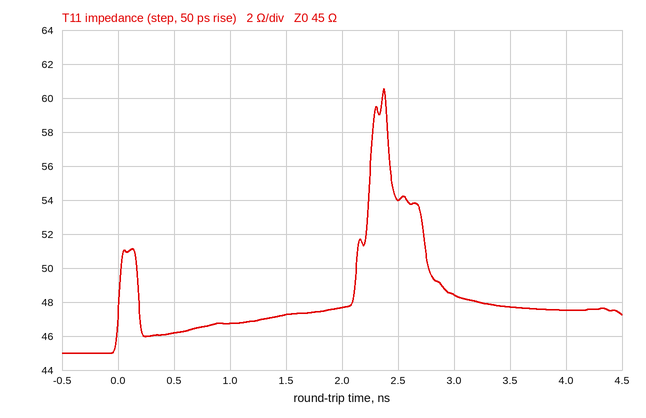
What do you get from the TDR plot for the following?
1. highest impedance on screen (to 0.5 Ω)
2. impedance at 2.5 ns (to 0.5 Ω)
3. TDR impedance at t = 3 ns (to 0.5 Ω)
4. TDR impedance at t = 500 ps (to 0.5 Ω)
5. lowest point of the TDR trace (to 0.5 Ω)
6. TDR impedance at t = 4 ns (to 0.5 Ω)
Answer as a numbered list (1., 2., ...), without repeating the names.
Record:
1. 60.5 Ω
2. 54.0 Ω
3. 48.5 Ω
4. 46.0 Ω
5. 45.0 Ω
6. 47.5 Ω
